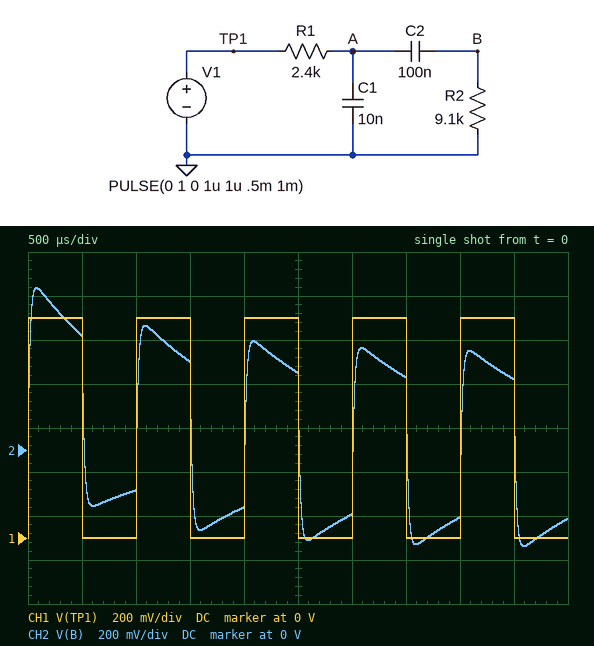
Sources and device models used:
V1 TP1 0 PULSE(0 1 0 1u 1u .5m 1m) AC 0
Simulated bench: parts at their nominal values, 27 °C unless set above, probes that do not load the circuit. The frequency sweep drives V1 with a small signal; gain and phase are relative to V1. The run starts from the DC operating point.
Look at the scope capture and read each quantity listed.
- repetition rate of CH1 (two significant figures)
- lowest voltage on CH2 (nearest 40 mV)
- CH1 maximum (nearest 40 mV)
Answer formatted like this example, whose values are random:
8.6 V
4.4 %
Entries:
1.0 kHz
-440 mV
1.00 V
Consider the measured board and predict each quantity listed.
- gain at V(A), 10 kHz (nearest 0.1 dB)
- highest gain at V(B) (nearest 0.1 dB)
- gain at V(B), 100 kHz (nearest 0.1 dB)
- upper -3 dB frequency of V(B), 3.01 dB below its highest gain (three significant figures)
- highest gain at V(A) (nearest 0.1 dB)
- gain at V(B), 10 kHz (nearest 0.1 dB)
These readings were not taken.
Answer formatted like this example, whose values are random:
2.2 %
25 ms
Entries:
-5.9 dB
-2.2 dB
-23.6 dB
8.69 kHz
0 dB
-5.9 dB
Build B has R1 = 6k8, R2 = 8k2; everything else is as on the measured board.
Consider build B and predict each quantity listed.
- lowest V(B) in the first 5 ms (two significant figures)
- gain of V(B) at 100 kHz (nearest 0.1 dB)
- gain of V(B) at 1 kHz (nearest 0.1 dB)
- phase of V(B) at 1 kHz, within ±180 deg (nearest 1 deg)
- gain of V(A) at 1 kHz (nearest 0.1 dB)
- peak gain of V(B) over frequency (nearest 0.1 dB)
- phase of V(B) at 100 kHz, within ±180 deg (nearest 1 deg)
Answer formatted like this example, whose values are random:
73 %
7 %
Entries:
-270 mV
-32.6 dB
-5.7 dB
-7 deg
-5.5 dB
-5.6 dB
-87 deg
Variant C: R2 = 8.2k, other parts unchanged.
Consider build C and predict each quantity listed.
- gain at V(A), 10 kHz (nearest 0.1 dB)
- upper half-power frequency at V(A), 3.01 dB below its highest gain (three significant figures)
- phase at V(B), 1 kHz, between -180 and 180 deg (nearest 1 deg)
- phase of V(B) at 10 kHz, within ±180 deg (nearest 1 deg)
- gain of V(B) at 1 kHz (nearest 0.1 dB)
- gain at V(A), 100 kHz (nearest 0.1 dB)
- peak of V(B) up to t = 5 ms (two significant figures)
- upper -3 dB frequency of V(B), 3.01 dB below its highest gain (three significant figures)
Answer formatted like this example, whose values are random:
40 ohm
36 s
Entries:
-6.0 dB
3.71 kHz
2 deg
-48 deg
-2.4 dB
-23.6 dB
720 mV
8.91 kHz
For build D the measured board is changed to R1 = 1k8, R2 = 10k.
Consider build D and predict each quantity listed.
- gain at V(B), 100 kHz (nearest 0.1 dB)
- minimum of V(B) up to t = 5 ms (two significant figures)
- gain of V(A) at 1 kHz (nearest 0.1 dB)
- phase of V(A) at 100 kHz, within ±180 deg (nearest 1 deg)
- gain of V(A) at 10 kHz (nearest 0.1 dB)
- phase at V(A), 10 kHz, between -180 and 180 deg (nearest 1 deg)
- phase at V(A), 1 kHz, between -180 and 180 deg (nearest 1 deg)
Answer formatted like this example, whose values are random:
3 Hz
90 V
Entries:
-21.1 dB
-470 mV
-1.5 dB
-84 deg
-4.3 dB
-44 deg
-7 deg
